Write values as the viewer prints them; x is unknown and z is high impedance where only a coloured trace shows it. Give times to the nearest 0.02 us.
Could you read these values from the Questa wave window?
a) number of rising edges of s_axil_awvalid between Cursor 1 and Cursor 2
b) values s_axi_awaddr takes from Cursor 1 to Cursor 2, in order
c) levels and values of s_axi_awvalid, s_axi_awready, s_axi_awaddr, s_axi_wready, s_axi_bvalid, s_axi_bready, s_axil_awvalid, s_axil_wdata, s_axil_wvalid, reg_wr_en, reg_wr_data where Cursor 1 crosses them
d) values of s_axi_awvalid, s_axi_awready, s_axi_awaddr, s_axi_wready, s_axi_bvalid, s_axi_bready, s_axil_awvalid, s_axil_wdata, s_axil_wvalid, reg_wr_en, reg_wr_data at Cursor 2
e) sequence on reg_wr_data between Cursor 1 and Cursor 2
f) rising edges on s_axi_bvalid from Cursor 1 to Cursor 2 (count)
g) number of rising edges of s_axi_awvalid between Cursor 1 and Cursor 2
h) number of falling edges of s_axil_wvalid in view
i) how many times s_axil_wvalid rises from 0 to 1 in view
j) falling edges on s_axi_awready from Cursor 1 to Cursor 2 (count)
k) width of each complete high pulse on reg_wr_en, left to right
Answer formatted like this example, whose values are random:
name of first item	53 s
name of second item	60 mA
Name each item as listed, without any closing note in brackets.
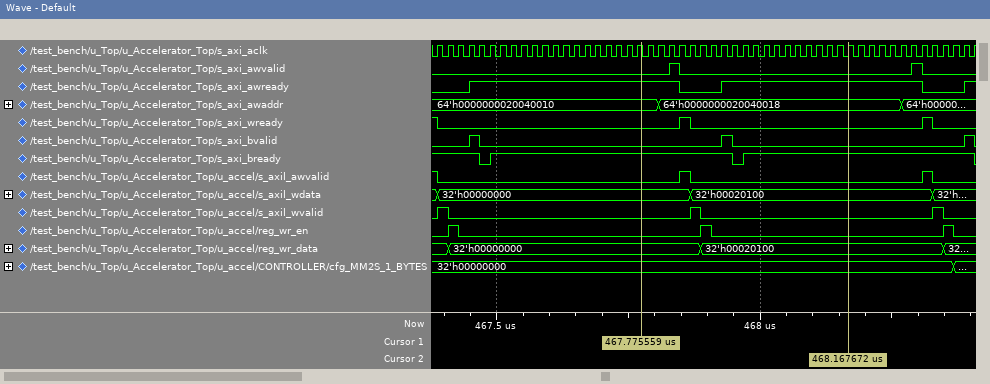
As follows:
number of rising edges of s_axil_awvalid between Cursor 1 and Cursor 2	1
values s_axi_awaddr takes from Cursor 1 to Cursor 2, in order	64'h0000000020040010, 64'h0000000020040018
levels and values of s_axi_awvalid, s_axi_awready, s_axi_awaddr, s_axi_wready, s_axi_bvalid, s_axi_bready, s_axil_awvalid, s_axil_wdata, s_axil_wvalid, reg_wr_en, reg_wr_data where Cursor 1 crosses them	s_axi_awvalid=0, s_axi_awready=1, s_axi_awaddr=64'h0000000020040010, s_axi_wready=0, s_axi_bvalid=0, s_axi_bready=1, s_axil_awvalid=0, s_axil_wdata=32'h00000000, s_axil_wvalid=0, reg_wr_en=0, reg_wr_data=32'h00000000
values of s_axi_awvalid, s_axi_awready, s_axi_awaddr, s_axi_wready, s_axi_bvalid, s_axi_bready, s_axil_awvalid, s_axil_wdata, s_axil_wvalid, reg_wr_en, reg_wr_data at Cursor 2	s_axi_awvalid=0, s_axi_awready=1, s_axi_awaddr=64'h0000000020040018, s_axi_wready=0, s_axi_bvalid=0, s_axi_bready=1, s_axil_awvalid=0, s_axil_wdata=32'h00020100, s_axil_wvalid=0, reg_wr_en=0, reg_wr_data=32'h00020100
sequence on reg_wr_data between Cursor 1 and Cursor 2	32'h00000000, 32'h00020100
rising edges on s_axi_bvalid from Cursor 1 to Cursor 2	1
number of rising edges of s_axi_awvalid between Cursor 1 and Cursor 2	1
number of falling edges of s_axil_wvalid in view	3
how many times s_axil_wvalid rises from 0 to 1 in view	3
falling edges on s_axi_awready from Cursor 1 to Cursor 2	1
width of each complete high pulse on reg_wr_en, left to right	0.02 us, 0.02 us, 0.02 us
